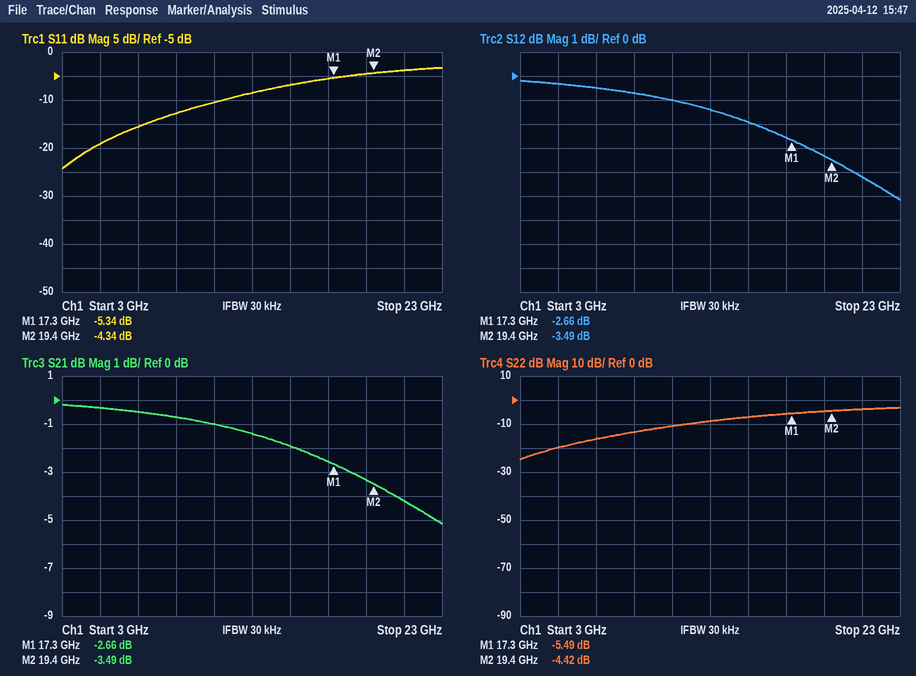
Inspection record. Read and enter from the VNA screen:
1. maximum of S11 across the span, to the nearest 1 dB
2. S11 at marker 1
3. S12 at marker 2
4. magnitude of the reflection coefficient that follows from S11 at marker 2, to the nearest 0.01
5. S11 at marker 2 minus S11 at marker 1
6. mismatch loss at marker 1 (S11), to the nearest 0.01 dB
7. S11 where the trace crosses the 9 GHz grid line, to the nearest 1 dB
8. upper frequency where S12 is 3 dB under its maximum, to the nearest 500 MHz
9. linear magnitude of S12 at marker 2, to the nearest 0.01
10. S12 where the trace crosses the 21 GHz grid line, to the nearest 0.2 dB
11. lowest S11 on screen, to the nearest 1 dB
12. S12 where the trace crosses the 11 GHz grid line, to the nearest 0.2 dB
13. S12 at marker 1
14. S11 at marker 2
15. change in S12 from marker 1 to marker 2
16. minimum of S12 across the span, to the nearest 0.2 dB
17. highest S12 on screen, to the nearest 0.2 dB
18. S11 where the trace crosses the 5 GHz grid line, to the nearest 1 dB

-3 dB
-5.34 dB
-3.49 dB
0.61
1.00 dB
1.50 dB
-13 dB
18.5 GHz
0.67
-4.2 dB
-24 dB
-1.0 dB
-2.66 dB
-4.34 dB
-0.83 dB
-5.2 dB
-0.2 dB
-19 dB
